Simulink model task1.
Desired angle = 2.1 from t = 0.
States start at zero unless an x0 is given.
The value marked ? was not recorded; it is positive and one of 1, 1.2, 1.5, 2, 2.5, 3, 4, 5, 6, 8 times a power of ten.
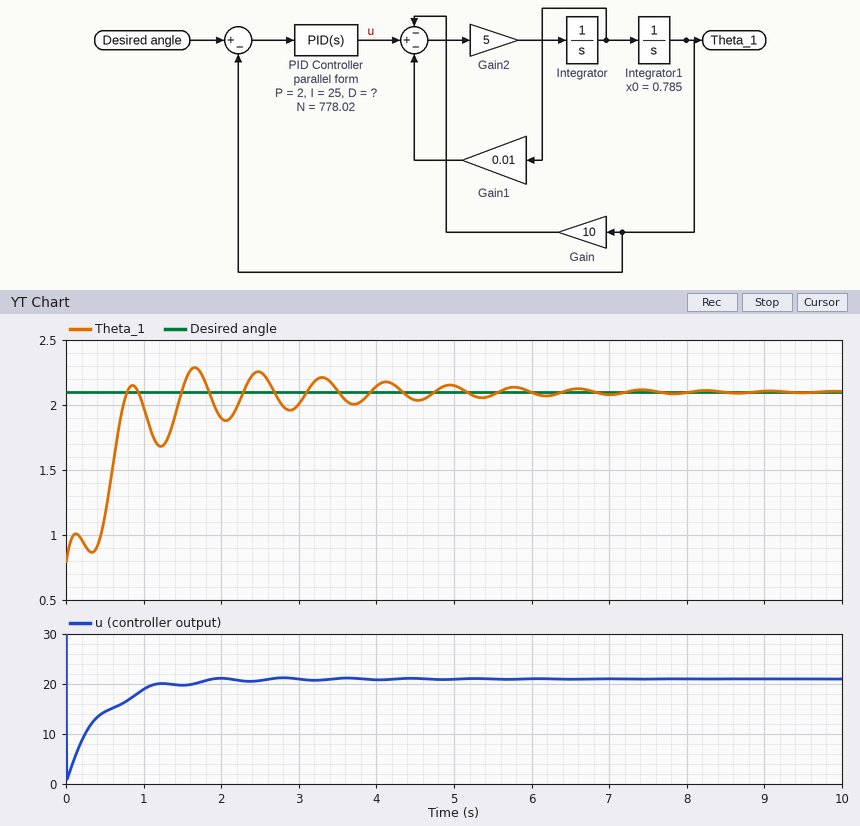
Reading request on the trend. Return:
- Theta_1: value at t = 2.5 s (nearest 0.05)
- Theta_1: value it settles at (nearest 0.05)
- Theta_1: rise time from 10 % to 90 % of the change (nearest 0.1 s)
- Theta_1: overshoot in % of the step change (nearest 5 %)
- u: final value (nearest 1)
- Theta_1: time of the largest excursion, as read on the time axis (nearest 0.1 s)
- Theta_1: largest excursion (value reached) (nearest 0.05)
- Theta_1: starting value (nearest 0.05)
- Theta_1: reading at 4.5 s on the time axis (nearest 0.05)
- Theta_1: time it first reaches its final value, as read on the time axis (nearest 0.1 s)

2.25
2.10
0.7 s
15 %
21
1.7 s
2.30
0.80
2.05
0.8 s
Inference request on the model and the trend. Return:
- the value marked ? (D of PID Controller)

0.6
